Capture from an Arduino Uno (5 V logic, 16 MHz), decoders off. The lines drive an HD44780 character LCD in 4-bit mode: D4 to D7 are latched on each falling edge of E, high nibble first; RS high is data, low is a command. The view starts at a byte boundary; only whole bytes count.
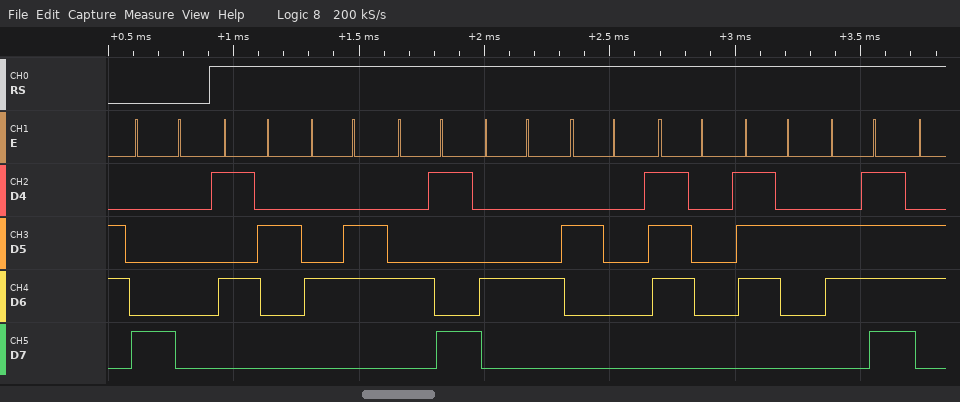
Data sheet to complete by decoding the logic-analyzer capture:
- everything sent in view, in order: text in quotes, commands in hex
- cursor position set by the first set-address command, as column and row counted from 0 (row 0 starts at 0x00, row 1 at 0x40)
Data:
0x80 "RFID pro"
column 0, row 0
